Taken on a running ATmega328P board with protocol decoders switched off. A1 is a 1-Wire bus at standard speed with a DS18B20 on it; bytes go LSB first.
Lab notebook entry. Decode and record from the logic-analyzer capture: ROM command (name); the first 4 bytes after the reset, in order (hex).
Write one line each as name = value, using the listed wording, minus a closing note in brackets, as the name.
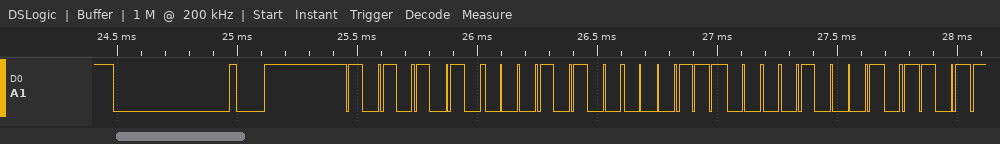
ROM command = Match ROM
the first 4 bytes after the reset, in order = 55 28 38 44
